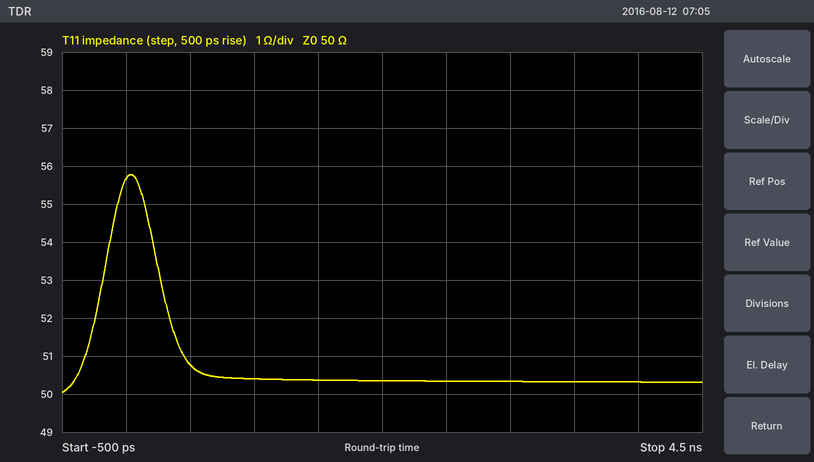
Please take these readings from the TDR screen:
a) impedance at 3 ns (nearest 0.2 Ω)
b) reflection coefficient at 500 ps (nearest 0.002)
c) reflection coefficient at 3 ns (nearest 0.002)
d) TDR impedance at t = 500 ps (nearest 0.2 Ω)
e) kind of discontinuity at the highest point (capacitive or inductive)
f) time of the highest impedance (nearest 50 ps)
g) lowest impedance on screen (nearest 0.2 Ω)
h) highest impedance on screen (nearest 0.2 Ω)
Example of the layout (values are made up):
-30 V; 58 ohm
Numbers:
50.4 Ω; +0.008; +0.004; 50.8 Ω; inductive; 50 ps; 50.0 Ω; 55.8 Ω
